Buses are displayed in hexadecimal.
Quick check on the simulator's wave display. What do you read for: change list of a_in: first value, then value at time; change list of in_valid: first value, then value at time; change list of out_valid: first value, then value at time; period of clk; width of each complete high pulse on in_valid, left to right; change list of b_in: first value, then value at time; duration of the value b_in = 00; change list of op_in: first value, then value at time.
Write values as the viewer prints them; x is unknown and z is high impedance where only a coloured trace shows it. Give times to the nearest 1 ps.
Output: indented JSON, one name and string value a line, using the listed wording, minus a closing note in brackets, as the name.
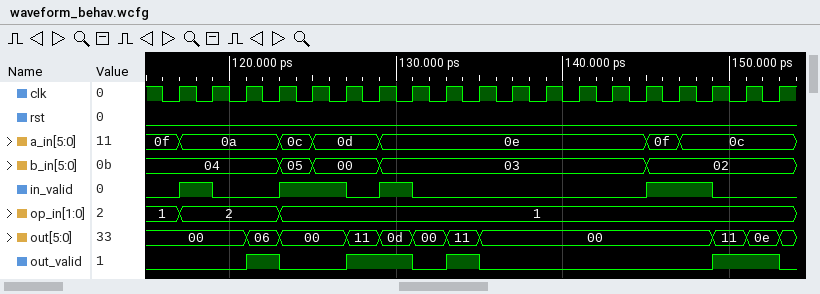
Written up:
{
  "change list of a_in: first value, then value at time": "0f, 0a at 117 ps, 0c at 123 ps, 0d at 125 ps, 0e at 129 ps, 0f at 145 ps, 0c at 147 ps",
  "change list of in_valid: first value, then value at time": "0, 1 at 117 ps, 0 at 119 ps, 1 at 123 ps, 0 at 127 ps, 1 at 129 ps, 0 at 131 ps, 1 at 145 ps, 0 at 149 ps",
  "change list of out_valid: first value, then value at time": "0, 1 at 121 ps, 0 at 123 ps, 1 at 127 ps, 0 at 131 ps, 1 at 133 ps, 0 at 135 ps, 1 at 149 ps, 0 at 153 ps",
  "period of clk": "2 ps",
  "width of each complete high pulse on in_valid, left to right": "2 ps, 4 ps, 2 ps, 4 ps",
  "change list of b_in: first value, then value at time": "04, 05 at 123 ps, 00 at 125 ps, 03 at 129 ps, 02 at 145 ps",
  "duration of the value b_in = 00": "4 ps",
  "change list of op_in: first value, then value at time": "1, 2 at 117 ps, 1 at 123 ps"
}
